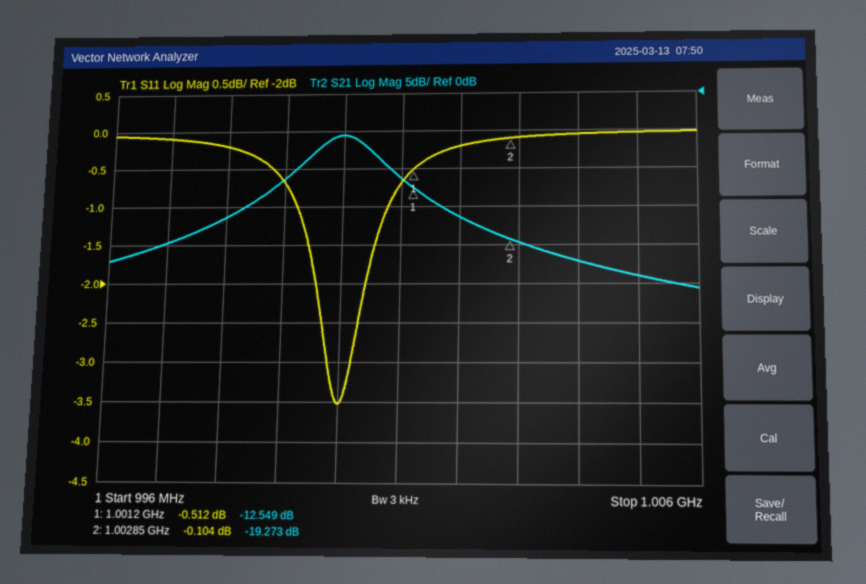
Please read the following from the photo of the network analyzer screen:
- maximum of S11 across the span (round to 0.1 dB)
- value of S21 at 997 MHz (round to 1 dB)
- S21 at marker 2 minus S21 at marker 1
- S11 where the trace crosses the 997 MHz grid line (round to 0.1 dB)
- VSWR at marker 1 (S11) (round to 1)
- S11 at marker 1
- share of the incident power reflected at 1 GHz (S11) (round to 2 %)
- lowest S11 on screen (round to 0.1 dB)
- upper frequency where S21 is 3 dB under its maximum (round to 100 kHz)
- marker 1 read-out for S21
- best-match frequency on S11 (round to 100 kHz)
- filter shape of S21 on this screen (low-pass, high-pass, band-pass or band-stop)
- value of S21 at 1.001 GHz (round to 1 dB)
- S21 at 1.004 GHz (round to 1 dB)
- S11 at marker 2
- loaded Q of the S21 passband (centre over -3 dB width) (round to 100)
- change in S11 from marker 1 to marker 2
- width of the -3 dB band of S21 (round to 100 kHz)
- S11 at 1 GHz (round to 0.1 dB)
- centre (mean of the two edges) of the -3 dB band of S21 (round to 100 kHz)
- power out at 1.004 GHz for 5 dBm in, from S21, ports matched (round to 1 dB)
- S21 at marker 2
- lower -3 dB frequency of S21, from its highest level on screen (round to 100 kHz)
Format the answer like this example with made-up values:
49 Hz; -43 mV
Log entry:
0.0 dB; -20 dB; -6.724 dB; -0.1 dB; 34; -0.512 dB; 44 %; -3.5 dB; 1.0006 GHz; -12.549 dB; 1.0000 GHz; band-pass; -11 dB; -22 dB; -0.104 dB; 800; 0.408 dB; 1.2 MHz; -3.5 dB; 1.0000 GHz; -17 dBm; -19.273 dB; 999.4 MHz
